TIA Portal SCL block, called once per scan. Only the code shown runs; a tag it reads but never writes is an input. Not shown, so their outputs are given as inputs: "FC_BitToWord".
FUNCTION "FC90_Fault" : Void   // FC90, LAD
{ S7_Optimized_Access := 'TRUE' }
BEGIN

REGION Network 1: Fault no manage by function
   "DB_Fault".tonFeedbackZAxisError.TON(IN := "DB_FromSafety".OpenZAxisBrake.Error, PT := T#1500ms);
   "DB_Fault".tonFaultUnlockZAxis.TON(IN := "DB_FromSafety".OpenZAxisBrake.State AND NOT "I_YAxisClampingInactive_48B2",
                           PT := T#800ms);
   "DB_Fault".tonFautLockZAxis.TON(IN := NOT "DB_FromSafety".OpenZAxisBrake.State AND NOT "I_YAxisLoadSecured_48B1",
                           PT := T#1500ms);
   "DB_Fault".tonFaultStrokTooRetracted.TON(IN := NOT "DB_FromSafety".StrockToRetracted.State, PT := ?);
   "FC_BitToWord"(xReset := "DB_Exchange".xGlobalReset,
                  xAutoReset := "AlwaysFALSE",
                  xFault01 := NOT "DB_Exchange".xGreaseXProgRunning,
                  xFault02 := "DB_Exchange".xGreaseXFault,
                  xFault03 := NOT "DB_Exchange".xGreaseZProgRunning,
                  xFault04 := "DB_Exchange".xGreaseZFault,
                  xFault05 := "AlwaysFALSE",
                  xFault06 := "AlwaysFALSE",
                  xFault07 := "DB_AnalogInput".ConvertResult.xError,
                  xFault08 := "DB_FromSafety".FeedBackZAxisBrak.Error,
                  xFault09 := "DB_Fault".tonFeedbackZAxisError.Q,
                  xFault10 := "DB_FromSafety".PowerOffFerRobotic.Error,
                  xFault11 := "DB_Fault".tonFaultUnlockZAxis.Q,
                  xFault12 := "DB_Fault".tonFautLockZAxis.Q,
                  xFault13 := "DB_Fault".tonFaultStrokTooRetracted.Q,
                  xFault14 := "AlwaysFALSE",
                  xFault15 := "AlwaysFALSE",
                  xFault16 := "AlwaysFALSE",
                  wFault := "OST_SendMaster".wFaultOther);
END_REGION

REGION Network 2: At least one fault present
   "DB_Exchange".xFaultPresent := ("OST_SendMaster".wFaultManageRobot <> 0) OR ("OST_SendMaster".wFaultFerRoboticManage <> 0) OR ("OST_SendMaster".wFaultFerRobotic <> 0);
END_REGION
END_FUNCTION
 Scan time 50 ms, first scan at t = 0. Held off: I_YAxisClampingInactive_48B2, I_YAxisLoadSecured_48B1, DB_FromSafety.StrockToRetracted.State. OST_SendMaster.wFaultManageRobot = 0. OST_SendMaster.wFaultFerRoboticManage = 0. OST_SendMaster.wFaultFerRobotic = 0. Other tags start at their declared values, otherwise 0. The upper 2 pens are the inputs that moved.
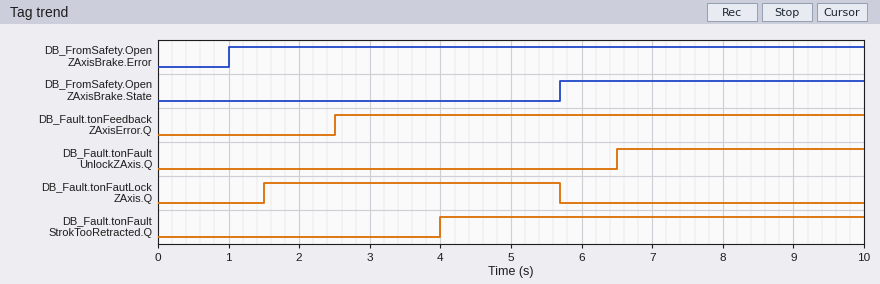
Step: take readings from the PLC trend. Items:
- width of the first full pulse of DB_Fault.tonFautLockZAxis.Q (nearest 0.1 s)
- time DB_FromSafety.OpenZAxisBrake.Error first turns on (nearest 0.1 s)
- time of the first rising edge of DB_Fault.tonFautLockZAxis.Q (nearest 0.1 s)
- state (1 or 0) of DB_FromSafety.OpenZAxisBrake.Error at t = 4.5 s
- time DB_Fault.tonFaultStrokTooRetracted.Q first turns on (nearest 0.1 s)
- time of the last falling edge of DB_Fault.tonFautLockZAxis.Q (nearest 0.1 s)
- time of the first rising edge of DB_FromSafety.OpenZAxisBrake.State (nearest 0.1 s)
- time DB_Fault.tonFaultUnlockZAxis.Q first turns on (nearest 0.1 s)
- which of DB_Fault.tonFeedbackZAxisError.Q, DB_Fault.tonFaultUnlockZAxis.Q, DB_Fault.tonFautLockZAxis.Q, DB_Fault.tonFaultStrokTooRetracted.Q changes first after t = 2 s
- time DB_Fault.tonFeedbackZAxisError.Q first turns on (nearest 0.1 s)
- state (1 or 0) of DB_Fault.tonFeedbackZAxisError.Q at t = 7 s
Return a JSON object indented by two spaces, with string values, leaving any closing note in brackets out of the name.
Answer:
{
  "width of the first full pulse of DB_Fault.tonFautLockZAxis.Q": "4.2 s",
  "time DB_FromSafety.OpenZAxisBrake.Error first turns on": "1.0 s",
  "time of the first rising edge of DB_Fault.tonFautLockZAxis.Q": "1.5 s",
  "state (1 or 0) of DB_FromSafety.OpenZAxisBrake.Error at t = 4.5 s": "1",
  "time DB_Fault.tonFaultStrokTooRetracted.Q first turns on": "4.0 s",
  "time of the last falling edge of DB_Fault.tonFautLockZAxis.Q": "5.7 s",
  "time of the first rising edge of DB_FromSafety.OpenZAxisBrake.State": "5.7 s",
  "time DB_Fault.tonFaultUnlockZAxis.Q first turns on": "6.5 s",
  "which of DB_Fault.tonFeedbackZAxisError.Q, DB_Fault.tonFaultUnlockZAxis.Q, DB_Fault.tonFautLockZAxis.Q, DB_Fault.tonFaultStrokTooRetracted.Q changes first after t = 2 s": "DB_Fault.tonFeedbackZAxisError.Q",
  "time DB_Fault.tonFeedbackZAxisError.Q first turns on": "2.5 s",
  "state (1 or 0) of DB_Fault.tonFeedbackZAxisError.Q at t = 7 s": "1"
}
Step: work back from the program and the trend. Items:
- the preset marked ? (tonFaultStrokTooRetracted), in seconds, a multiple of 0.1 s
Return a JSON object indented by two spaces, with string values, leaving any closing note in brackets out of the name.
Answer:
{
  "the preset marked ? (tonFaultStrokTooRetracted), in seconds, a multiple of 0.1 s": "4.0 s"
}
